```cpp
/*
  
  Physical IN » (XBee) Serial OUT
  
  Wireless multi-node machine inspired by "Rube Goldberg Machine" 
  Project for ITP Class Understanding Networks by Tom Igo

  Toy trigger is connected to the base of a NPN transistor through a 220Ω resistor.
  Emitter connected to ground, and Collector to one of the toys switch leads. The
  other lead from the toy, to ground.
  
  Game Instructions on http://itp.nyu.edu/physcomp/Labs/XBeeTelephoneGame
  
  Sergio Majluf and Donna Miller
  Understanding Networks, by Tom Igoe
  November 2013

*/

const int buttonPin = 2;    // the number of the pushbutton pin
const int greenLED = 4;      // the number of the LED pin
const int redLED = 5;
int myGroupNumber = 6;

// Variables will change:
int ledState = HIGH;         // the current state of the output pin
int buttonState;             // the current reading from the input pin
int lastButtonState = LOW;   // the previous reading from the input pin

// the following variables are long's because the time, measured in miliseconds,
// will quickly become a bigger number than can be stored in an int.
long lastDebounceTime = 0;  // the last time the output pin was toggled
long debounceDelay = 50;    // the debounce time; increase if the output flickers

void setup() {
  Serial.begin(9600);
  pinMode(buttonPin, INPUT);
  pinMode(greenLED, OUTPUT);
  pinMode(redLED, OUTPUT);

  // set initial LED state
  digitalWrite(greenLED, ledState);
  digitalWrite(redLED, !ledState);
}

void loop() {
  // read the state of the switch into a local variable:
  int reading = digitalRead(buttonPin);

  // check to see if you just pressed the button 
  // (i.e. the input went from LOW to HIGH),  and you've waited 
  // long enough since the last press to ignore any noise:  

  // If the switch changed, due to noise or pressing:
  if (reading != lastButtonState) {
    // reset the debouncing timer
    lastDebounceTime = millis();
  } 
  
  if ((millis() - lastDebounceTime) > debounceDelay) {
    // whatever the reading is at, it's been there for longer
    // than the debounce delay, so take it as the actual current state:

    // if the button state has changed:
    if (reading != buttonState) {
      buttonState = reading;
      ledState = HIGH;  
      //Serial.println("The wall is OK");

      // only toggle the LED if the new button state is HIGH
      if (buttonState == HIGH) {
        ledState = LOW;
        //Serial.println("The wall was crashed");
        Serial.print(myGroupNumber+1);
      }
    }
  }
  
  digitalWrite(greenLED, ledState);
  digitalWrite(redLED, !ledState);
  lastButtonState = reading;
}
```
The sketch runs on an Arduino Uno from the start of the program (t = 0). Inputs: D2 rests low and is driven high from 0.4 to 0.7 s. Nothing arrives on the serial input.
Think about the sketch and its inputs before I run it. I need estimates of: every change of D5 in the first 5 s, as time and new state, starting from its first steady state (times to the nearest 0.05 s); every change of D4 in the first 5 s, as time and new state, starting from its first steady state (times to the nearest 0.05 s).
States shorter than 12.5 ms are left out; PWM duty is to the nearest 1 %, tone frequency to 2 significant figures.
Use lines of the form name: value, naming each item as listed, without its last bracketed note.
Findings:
every change of D5 in the first 5 s, as time and new state, starting from its first steady state: 0 s low; 0.45 s high; 0.75 s low
every change of D4 in the first 5 s, as time and new state, starting from its first steady state: 0 s high; 0.45 s low; 0.75 s high
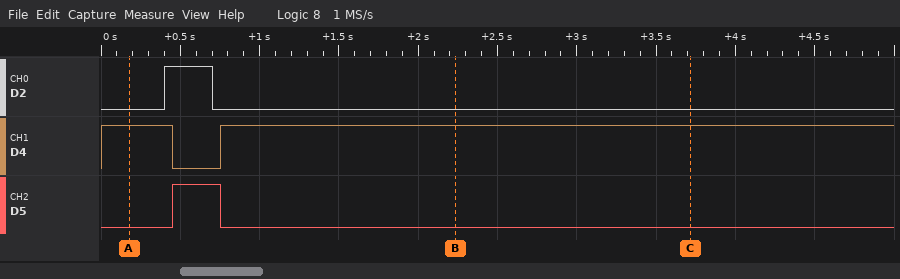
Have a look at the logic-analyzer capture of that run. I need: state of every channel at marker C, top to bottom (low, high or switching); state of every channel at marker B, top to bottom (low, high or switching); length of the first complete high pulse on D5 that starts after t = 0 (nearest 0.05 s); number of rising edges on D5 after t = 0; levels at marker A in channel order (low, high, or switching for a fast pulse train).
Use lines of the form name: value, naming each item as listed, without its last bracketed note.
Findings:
state of every channel at marker C, top to bottom: D2 low, D4 high, D5 low
state of every channel at marker B, top to bottom: D2 low, D4 high, D5 low
length of the first complete high pulse on D5 that starts after t = 0: 0.30 s
number of rising edges on D5 after t = 0: 1
levels at marker A in channel order: D2 low, D4 high, D5 low
